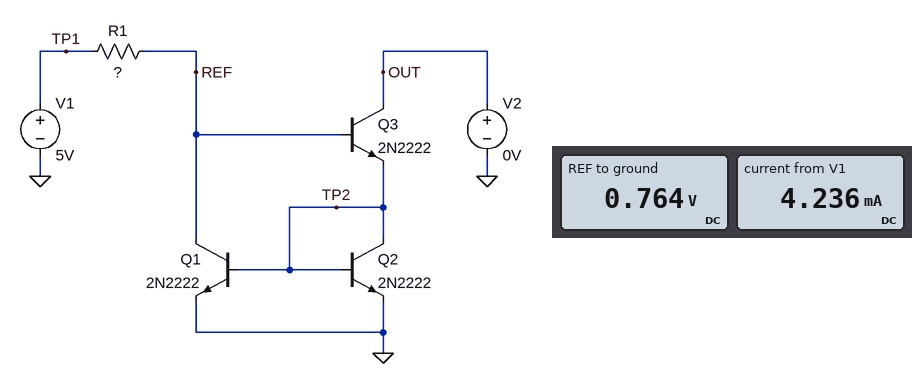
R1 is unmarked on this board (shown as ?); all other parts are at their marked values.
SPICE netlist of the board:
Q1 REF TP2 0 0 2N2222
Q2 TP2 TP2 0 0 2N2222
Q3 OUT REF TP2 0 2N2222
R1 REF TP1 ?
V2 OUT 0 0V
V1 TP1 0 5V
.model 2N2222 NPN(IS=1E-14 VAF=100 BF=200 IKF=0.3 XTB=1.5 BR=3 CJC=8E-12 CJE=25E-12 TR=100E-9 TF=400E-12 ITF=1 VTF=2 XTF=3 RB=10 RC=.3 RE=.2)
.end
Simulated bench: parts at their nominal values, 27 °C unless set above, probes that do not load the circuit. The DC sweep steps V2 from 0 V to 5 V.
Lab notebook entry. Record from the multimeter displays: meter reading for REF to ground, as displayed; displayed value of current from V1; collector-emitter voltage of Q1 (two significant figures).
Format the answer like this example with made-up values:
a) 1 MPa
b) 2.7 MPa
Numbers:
a) 0.764 V
b) 4.236 mA
c) 760 mV
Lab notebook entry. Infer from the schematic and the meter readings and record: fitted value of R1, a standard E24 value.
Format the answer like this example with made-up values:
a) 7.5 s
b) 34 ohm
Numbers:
a) 1 kΩ
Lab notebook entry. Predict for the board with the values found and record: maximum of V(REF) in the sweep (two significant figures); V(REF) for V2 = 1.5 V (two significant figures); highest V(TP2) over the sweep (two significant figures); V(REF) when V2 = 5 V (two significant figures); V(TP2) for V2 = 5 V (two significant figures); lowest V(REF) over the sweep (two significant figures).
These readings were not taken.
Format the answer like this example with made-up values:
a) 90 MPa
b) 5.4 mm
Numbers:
a) 1.4 V
b) 1.4 V
c) 690 mV
d) 1.4 V
e) 690 mV
f) 760 mV
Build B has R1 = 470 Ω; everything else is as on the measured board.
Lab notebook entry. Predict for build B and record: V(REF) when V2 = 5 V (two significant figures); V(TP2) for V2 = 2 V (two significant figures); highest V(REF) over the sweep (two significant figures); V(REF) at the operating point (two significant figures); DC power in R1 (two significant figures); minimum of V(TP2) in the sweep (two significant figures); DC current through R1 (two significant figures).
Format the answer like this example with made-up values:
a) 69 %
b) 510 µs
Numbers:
a) 1.4 V
b) 710 mV
c) 1.5 V
d) 830 mV
e) 37 mW
f) 2.8 mV
g) 8.9 mA
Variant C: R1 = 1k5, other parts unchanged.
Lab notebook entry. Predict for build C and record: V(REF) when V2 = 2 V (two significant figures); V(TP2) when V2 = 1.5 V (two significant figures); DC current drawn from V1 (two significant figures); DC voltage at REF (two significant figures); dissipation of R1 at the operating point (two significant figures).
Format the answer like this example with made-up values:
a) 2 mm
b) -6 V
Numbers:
a) 1.4 V
b) 680 mV
c) 2.8 mA
d) 740 mV
e) 12 mW
